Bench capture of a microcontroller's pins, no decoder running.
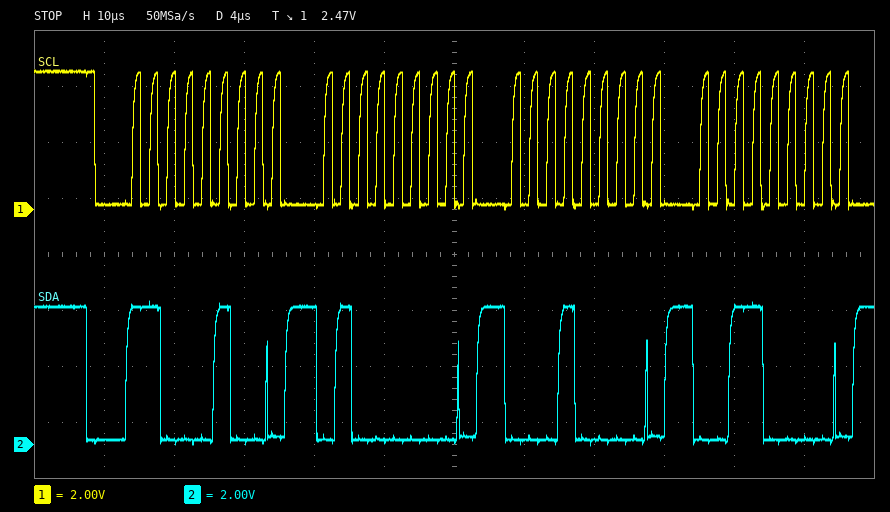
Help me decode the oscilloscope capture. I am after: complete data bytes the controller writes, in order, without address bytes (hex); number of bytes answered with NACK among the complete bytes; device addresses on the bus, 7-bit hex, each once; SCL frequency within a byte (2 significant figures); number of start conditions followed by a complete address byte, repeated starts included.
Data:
40 10 30
0
0x62
400 kHz
1
